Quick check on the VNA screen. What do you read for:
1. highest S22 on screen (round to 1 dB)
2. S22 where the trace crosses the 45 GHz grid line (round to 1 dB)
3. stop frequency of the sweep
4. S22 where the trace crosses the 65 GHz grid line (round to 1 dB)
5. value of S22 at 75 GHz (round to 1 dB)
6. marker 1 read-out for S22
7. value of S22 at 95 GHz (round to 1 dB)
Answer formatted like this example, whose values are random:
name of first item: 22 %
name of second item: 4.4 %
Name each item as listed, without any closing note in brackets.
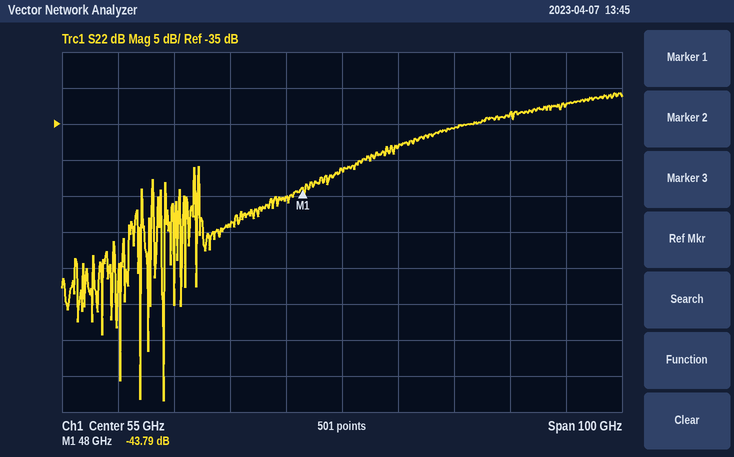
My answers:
highest S22 on screen: -31 dB
S22 where the trace crosses the 45 GHz grid line: -45 dB
stop frequency of the sweep: 105 GHz
S22 where the trace crosses the 65 GHz grid line: -38 dB
value of S22 at 75 GHz: -36 dB
marker 1 read-out for S22: -43.79 dB
value of S22 at 95 GHz: -32 dB
